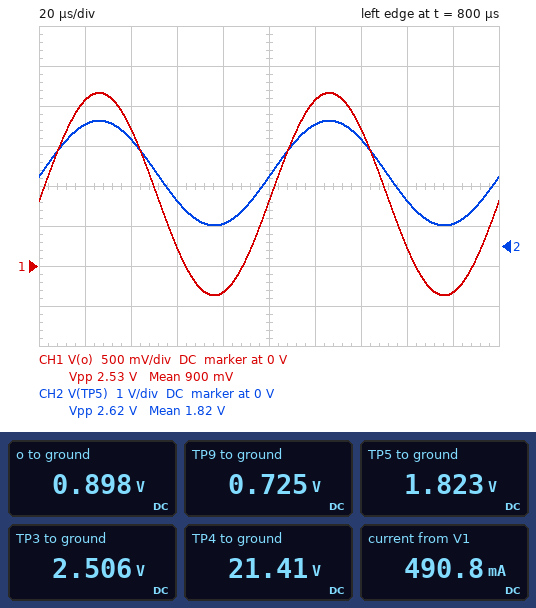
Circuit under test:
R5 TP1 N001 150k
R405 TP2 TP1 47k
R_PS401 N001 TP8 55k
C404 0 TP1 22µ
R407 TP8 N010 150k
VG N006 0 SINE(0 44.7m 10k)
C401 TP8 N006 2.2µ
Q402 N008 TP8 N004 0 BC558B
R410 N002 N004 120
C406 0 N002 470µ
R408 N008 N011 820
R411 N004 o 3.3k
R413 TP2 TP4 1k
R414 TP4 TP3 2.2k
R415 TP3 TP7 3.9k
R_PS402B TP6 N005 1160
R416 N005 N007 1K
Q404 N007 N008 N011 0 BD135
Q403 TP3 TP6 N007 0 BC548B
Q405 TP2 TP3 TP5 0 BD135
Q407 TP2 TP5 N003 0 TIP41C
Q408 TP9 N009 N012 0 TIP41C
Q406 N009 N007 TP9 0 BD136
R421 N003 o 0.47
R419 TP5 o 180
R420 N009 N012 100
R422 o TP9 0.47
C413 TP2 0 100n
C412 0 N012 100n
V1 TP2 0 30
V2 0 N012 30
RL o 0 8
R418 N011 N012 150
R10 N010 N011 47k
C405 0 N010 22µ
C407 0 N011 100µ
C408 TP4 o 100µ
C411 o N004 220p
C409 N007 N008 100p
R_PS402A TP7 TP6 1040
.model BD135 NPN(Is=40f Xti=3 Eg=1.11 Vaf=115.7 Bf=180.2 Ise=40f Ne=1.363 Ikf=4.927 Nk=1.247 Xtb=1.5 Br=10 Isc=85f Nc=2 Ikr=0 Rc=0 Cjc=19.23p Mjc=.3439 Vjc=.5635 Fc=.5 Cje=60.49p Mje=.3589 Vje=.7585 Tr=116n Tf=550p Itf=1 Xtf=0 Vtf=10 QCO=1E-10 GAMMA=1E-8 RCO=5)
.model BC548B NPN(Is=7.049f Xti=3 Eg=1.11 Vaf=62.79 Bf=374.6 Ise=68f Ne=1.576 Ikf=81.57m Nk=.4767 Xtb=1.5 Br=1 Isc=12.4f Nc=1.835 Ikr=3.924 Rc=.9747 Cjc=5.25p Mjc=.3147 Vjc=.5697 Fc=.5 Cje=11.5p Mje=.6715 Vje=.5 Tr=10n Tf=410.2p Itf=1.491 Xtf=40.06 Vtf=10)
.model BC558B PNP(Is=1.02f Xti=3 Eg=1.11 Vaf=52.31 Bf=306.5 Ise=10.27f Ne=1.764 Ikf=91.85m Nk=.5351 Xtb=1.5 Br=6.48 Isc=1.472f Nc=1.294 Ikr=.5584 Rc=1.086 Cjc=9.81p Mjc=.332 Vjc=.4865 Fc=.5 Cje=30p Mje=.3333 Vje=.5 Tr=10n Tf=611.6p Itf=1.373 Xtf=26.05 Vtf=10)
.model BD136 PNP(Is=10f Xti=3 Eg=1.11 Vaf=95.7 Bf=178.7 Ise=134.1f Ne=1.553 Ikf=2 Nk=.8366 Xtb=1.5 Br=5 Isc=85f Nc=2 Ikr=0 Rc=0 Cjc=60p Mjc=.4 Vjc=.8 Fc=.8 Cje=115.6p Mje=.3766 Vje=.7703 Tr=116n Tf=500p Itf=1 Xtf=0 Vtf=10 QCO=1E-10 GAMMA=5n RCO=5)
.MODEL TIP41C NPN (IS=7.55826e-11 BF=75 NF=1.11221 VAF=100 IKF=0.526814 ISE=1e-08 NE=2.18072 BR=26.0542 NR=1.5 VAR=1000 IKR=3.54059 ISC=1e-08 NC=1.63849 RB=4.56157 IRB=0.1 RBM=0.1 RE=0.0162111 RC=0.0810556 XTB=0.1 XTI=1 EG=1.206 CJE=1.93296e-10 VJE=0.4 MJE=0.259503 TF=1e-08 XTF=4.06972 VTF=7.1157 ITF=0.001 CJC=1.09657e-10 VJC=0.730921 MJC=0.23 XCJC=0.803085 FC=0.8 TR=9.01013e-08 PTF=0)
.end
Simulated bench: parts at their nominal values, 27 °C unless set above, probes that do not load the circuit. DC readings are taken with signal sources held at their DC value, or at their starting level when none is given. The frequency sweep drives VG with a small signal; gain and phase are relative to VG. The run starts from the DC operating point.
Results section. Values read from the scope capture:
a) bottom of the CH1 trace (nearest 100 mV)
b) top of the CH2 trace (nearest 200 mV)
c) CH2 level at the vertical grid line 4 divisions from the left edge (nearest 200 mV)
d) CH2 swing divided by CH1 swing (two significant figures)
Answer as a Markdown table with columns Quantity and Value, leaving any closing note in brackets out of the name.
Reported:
| Quantity | Value |
|---|---|
| bottom of the CH1 trace | -400 mV |
| top of the CH2 trace | 3.2 V |
| CH2 level at the vertical grid line 4 divisions from the left edge | 600 mV |
| CH2 swing divided by CH1 swing | 1.0 |
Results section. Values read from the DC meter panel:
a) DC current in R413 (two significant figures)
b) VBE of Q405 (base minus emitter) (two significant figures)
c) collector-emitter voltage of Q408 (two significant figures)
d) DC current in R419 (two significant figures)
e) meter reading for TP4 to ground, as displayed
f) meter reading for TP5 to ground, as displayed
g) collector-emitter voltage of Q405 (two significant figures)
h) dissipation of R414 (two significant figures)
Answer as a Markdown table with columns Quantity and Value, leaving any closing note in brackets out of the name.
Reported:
| Quantity | Value |
|---|---|
| DC current in R413 | 8.6 mA |
| VBE of Q405 (base minus emitter) | 680 mV |
| collector-emitter voltage of Q408 | 31 V |
| DC current in R419 | 5.1 mA |
| meter reading for TP4 to ground, as displayed | 21.41 V |
| meter reading for TP5 to ground, as displayed | 1.823 V |
| collector-emitter voltage of Q405 | 28 V |
| dissipation of R414 | 160 mW |
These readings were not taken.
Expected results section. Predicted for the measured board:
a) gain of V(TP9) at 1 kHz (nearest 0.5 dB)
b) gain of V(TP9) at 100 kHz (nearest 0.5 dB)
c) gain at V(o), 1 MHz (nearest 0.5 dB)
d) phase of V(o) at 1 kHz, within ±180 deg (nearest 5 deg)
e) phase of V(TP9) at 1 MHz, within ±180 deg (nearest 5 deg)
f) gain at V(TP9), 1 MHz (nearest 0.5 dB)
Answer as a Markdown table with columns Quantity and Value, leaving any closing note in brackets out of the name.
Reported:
| Quantity | Value |
|---|---|
| gain of V(TP9) at 1 kHz | 29.5 dB |
| gain of V(TP9) at 100 kHz | 27.5 dB |
| gain at V(o), 1 MHz | 11.5 dB |
| phase of V(o) at 1 kHz, within ±180 deg | 0 deg |
| phase of V(TP9) at 1 MHz, within ±180 deg | -75 deg |
| gain at V(TP9), 1 MHz | 12.0 dB |
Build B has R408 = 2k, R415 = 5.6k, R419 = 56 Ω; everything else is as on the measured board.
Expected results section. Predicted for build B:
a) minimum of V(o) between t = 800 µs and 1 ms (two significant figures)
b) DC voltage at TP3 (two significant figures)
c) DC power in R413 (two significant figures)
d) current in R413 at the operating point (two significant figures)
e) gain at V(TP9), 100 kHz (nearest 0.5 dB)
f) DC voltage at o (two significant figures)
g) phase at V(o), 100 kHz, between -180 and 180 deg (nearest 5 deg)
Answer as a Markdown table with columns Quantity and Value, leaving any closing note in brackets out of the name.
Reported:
| Quantity | Value |
|---|---|
| minimum of V(o) between t = 800 µs and 1 ms | -2.1 V |
| DC voltage at TP3 | 1.1 V |
| DC power in R413 | 82 mW |
| current in R413 at the operating point | 9.0 mA |
| gain at V(TP9), 100 kHz | 27.0 dB |
| DC voltage at o | -830 mV |
| phase at V(o), 100 kHz, between -180 and 180 deg | -40 deg |
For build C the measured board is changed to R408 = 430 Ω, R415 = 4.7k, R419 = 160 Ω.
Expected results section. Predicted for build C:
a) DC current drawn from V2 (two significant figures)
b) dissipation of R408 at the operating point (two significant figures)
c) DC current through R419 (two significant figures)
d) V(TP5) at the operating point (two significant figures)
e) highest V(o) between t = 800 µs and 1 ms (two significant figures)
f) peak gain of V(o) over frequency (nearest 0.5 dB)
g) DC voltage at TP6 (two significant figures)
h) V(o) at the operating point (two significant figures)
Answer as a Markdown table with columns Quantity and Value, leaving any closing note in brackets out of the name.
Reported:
| Quantity | Value |
|---|---|
| DC current drawn from V2 | 400 mA |
| dissipation of R408 at the operating point | 1.0 mW |
| DC current through R419 | 7.2 mA |
| V(TP5) at the operating point | 4.6 V |
| highest V(o) between t = 800 µs and 1 ms | 4.7 V |
| peak gain of V(o) over frequency | 29.0 dB |
| DC voltage at TP6 | 3.3 V |
| V(o) at the operating point | 3.5 V |
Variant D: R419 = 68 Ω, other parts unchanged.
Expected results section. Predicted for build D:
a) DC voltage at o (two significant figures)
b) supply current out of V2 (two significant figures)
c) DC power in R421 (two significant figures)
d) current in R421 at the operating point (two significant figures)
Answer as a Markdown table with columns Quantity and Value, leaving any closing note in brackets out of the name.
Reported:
| Quantity | Value |
|---|---|
| DC voltage at o | 890 mV |
| supply current out of V2 | 370 mA |
| DC power in R421 | 100 mW |
| current in R421 at the operating point | 460 mA |
